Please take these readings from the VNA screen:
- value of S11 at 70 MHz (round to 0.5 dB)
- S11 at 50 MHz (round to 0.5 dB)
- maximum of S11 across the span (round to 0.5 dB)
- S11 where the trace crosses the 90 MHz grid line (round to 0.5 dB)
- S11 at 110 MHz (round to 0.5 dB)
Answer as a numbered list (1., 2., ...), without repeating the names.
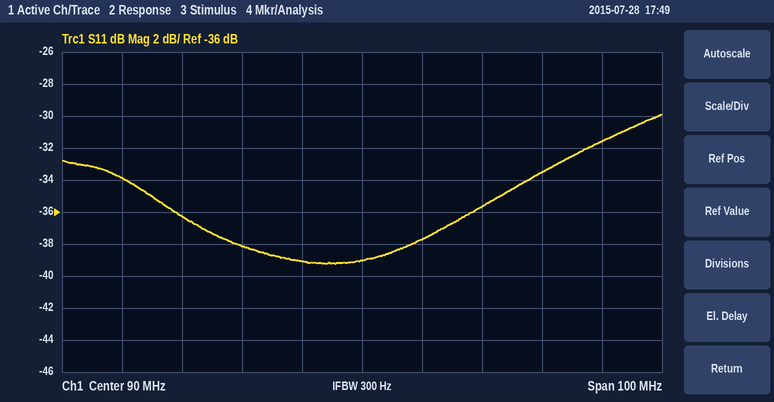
1. -38.0 dB
2. -34.0 dB
3. -30.0 dB
4. -39.0 dB
5. -35.5 dB
